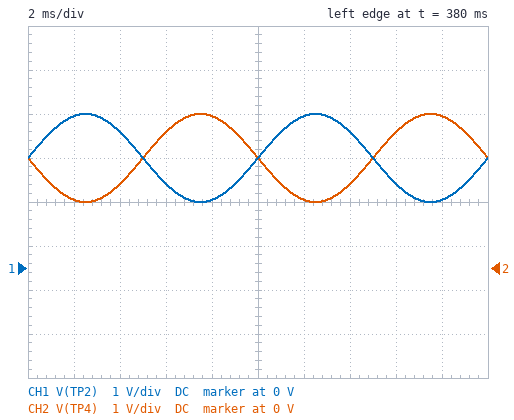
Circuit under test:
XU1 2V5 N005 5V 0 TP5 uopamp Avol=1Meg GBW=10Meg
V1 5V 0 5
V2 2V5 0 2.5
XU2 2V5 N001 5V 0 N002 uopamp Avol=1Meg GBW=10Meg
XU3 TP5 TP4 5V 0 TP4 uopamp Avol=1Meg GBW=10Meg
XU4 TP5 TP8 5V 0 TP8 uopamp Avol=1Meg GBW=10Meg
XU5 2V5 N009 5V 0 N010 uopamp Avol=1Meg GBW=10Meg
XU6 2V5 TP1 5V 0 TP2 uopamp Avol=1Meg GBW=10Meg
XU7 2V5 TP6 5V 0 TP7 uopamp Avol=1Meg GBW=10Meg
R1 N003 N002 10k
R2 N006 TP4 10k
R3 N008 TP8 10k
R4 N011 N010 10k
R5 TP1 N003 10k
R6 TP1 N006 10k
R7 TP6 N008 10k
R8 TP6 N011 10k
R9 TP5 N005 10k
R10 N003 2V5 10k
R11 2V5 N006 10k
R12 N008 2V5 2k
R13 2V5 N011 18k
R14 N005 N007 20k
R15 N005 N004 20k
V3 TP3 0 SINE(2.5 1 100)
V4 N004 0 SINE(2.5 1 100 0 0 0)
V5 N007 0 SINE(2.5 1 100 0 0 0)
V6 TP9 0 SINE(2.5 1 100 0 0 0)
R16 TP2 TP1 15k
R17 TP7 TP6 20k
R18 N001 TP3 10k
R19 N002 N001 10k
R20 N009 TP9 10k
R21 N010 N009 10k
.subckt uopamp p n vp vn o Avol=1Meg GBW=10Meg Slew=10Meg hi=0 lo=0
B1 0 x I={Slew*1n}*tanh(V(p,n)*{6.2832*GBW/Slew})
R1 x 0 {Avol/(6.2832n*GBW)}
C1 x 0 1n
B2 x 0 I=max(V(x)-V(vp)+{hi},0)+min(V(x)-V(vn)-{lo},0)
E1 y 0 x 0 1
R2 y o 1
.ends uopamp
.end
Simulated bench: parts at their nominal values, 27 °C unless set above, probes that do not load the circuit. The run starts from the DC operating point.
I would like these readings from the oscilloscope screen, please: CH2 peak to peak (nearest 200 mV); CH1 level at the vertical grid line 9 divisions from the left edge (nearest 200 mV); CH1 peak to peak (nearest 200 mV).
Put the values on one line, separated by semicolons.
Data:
2.0 V; 1.6 V; 2.0 V
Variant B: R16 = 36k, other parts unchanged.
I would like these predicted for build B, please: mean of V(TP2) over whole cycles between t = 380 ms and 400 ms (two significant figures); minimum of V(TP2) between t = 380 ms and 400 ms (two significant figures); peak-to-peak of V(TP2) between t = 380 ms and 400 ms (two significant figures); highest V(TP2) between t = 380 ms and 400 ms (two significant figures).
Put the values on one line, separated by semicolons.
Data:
2.5 V; 100 mV; 4.8 V; 4.9 V
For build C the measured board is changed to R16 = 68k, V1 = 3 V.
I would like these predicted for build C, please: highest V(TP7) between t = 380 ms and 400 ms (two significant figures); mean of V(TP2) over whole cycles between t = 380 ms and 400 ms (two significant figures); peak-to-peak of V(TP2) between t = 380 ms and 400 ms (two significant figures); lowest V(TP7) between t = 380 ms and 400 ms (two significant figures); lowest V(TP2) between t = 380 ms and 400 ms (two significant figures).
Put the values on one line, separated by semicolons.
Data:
3.0 V; 1.8 V; 2.8 V; 2.0 V; 210 mV
